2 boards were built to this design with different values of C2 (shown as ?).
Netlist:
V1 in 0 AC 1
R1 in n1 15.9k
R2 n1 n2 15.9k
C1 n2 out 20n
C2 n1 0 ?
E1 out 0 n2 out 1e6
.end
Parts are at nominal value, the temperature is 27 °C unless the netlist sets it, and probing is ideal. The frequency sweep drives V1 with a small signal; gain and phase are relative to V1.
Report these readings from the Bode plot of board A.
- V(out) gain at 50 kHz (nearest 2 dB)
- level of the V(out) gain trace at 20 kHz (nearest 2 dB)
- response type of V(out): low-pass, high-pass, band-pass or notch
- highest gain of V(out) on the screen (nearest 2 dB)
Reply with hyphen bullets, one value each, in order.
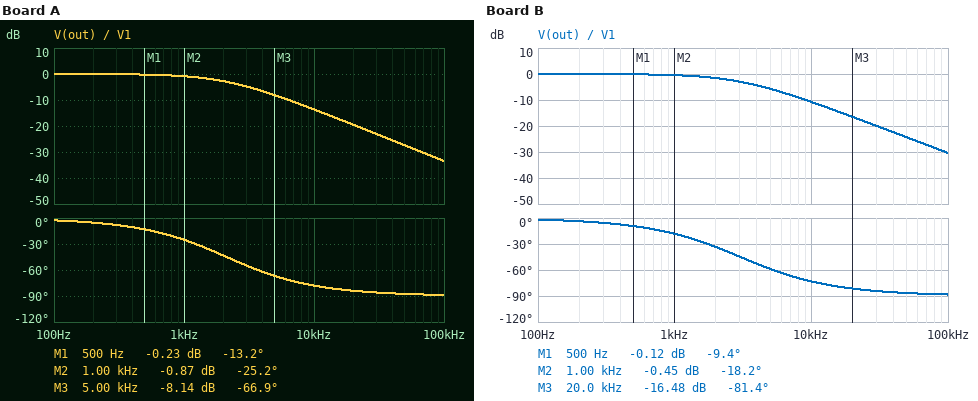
- -28 dB
- -20 dB
- low-pass
- 0 dB
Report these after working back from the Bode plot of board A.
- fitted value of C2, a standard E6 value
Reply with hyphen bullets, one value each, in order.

- 4.7 nF
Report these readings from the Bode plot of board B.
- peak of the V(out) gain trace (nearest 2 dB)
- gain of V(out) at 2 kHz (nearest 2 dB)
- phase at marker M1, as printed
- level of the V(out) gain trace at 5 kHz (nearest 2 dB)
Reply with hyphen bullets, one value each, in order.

- 0 dB
- -2 dB
- -9.4 deg
- -6 dB
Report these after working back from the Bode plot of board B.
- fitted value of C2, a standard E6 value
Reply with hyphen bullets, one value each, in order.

- 3.3 nF
